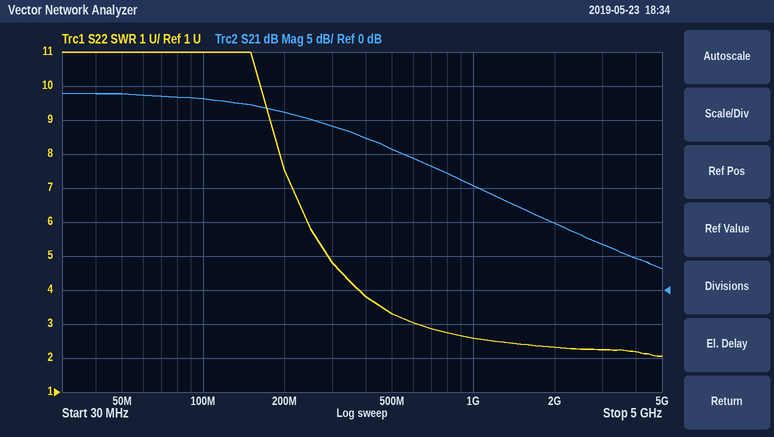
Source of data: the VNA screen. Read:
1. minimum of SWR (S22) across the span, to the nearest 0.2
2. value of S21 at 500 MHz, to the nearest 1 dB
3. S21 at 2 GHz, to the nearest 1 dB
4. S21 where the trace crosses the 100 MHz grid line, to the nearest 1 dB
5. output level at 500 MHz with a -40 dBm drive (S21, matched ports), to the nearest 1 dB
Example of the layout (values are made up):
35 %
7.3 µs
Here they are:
2.0
21 dB
10 dB
28 dB
-19 dBm
